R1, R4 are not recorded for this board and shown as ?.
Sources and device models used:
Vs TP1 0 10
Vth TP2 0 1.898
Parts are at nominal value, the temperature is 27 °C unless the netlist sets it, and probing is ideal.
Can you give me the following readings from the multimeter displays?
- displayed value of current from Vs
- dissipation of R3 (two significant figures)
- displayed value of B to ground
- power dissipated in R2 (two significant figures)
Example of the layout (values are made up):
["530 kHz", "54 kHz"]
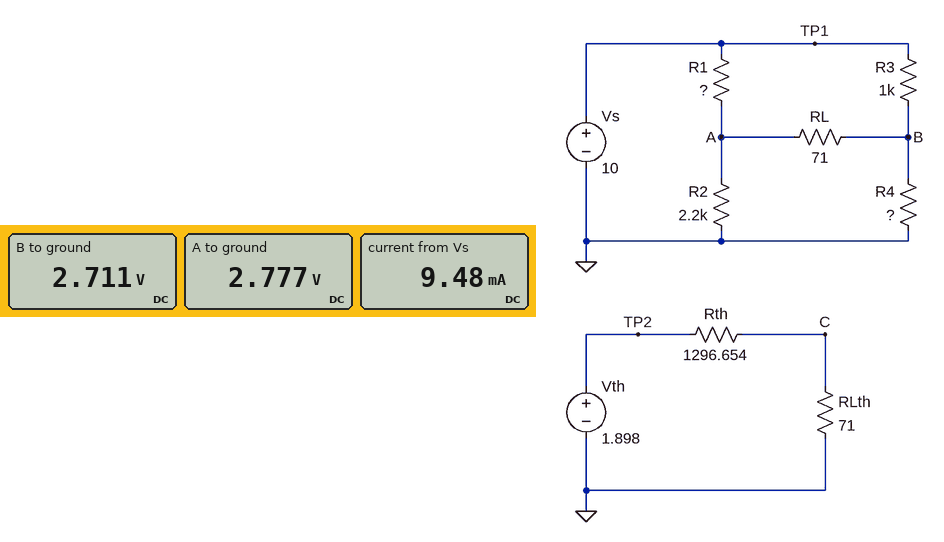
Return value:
["9.48 mA", "53 mW", "2.711 V", "3.5 mW"]
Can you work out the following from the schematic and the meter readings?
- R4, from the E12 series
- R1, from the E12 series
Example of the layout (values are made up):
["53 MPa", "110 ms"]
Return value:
["330 Ω", "3.3 kΩ"]
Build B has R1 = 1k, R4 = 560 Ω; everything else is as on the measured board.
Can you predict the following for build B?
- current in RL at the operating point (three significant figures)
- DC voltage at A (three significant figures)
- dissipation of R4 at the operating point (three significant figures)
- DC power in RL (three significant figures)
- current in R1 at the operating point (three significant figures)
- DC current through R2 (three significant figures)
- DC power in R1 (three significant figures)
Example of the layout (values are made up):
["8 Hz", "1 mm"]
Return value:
["2.94 mA", "4.85 V", "38.5 mW", "614 µW", "5.15 mA", "2.21 mA", "26.5 mW"]
